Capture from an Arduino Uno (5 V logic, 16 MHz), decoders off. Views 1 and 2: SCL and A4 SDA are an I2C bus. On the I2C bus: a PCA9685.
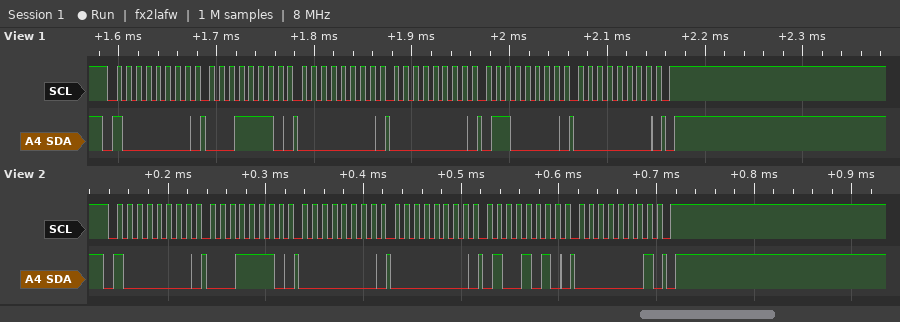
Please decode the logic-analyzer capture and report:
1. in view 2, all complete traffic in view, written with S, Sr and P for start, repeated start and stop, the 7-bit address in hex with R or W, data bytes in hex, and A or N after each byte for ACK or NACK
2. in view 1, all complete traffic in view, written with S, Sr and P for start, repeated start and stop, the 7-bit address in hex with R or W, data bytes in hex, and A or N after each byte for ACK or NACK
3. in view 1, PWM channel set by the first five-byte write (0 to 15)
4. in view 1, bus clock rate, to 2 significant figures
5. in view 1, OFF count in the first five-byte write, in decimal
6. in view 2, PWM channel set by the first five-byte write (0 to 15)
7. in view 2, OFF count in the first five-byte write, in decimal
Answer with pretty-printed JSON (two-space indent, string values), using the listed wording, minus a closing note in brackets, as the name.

{
  "in view 2, all complete traffic in view, written with S, Sr and P for start, repeated start and stop, the 7-bit address in hex with R or W, data bytes in hex, and A or N after each byte for ACK or NACK": "S 40W A 1E A 00 A 00 A 4A A 01 A P",
  "in view 1, all complete traffic in view, written with S, Sr and P for start, repeated start and stop, the 7-bit address in hex with R or W, data bytes in hex, and A or N after each byte for ACK or NACK": "S 40W A 1E A 00 A 00 A 60 A 00 A P",
  "in view 1, PWM channel set by the first five-byte write": "6",
  "in view 1, bus clock rate, to 2 significant figures": "100 kHz",
  "in view 1, OFF count in the first five-byte write, in decimal": "96",
  "in view 2, PWM channel set by the first five-byte write": "6",
  "in view 2, OFF count in the first five-byte write, in decimal": "330"
}
